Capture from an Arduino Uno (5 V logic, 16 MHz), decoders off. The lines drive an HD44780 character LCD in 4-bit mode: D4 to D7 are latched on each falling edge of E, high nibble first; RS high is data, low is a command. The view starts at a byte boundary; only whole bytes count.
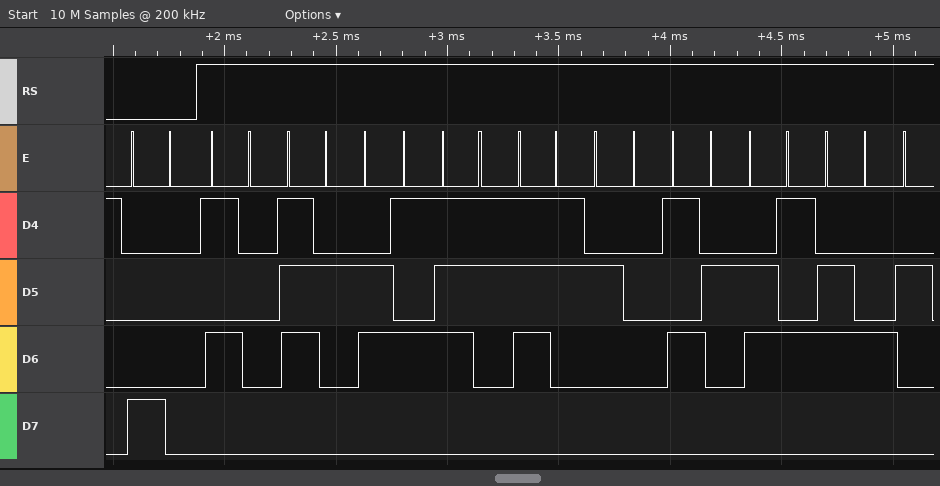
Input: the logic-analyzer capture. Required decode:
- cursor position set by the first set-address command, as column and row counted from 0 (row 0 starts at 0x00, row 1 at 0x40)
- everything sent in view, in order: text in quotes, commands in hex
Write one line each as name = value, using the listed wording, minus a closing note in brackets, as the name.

cursor position set by the first set-address command, as column and row counted from 0 = column 0, row 0
everything sent in view, in order: text in quotes, commands in hex = 0x80 "Press Red"
